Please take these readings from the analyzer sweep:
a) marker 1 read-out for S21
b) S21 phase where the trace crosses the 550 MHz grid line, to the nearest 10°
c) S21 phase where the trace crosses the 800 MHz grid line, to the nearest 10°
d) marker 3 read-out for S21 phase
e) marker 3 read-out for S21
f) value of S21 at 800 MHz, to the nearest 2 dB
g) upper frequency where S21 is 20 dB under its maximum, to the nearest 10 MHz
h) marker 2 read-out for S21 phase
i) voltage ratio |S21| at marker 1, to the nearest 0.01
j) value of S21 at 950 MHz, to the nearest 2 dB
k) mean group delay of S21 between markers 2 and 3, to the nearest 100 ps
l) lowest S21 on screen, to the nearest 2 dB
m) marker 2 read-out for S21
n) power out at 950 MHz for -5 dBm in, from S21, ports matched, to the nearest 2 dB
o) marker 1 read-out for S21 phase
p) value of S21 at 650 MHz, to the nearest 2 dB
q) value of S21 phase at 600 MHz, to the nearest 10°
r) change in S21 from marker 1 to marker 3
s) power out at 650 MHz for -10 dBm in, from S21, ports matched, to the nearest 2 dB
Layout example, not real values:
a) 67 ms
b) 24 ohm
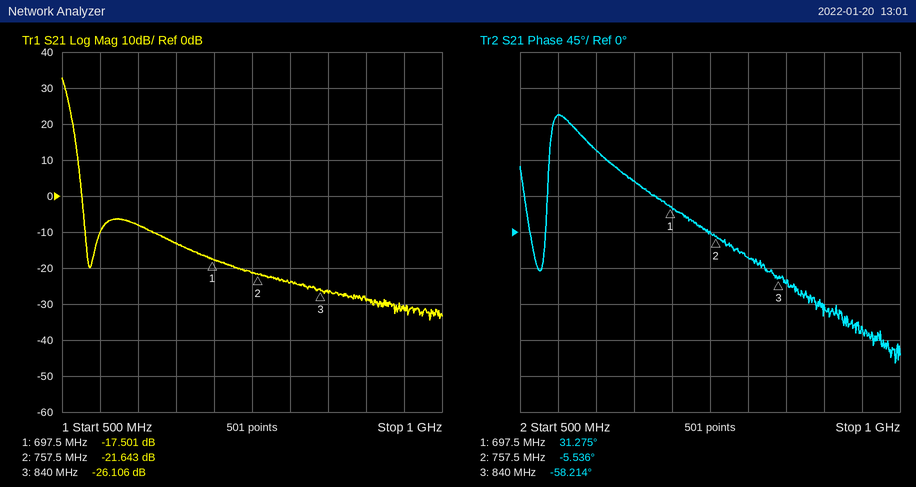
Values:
a) -17.501 dB
b) 150°
c) -30°
d) -58.214°
e) -26.106 dB
f) -24 dB
g) 520 MHz
h) -5.536°
i) 0.13
j) -32 dB
k) 1.8 ns
l) -34 dB
m) -21.643 dB
n) -36 dBm
o) 31.275°
p) -14 dB
q) 100°
r) -8.605 dB
s) -24 dBm
